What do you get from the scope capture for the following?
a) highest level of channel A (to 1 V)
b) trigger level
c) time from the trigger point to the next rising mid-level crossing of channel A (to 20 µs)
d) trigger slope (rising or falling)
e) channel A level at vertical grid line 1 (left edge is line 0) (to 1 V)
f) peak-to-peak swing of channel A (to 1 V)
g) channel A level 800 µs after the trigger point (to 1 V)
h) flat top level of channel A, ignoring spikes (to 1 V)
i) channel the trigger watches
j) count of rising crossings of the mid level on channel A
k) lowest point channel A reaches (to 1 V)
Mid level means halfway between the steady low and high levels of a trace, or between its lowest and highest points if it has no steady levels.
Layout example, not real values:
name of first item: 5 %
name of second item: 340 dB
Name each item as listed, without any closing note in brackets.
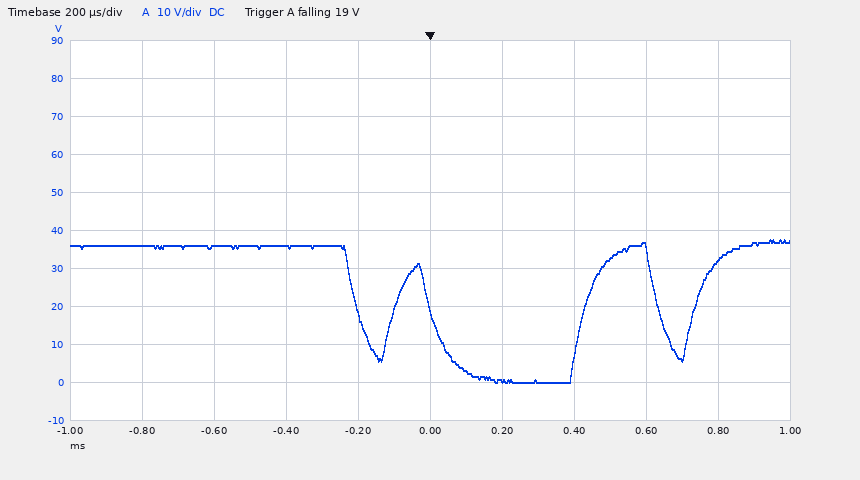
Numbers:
highest level of channel A: 38 V
trigger level: 19 V
time from the trigger point to the next rising mid-level crossing of channel A: 420 µs
trigger slope: falling
channel A level at vertical grid line 1 (left edge is line 0): 36 V
peak-to-peak swing of channel A: 38 V
channel A level 800 µs after the trigger point: 32 V
flat top level of channel A, ignoring spikes: 36 V
channel the trigger watches: channel A
count of rising crossings of the mid level on channel A: 3
lowest point channel A reaches: 0 V
